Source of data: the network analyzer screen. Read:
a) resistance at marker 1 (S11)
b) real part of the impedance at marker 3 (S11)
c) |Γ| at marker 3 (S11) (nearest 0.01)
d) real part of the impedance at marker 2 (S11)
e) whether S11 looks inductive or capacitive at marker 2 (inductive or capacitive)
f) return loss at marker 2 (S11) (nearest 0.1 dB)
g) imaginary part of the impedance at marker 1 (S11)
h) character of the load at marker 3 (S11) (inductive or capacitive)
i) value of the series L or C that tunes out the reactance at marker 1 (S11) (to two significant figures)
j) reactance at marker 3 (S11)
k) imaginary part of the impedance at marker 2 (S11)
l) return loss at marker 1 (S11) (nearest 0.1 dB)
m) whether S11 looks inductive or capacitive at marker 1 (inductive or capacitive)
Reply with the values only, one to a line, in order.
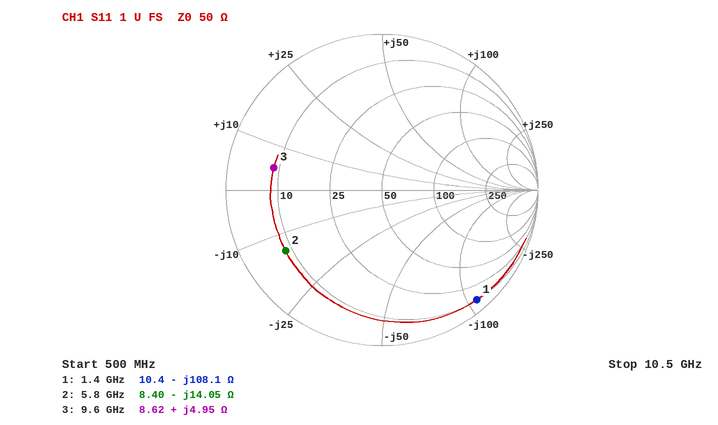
10.4 Ω
8.62 Ω
0.71
8.40 Ω
capacitive
2.7 dB
-108.1 Ω
inductive
12 nH
+4.95 Ω
-14.05 Ω
0.6 dB
capacitive
